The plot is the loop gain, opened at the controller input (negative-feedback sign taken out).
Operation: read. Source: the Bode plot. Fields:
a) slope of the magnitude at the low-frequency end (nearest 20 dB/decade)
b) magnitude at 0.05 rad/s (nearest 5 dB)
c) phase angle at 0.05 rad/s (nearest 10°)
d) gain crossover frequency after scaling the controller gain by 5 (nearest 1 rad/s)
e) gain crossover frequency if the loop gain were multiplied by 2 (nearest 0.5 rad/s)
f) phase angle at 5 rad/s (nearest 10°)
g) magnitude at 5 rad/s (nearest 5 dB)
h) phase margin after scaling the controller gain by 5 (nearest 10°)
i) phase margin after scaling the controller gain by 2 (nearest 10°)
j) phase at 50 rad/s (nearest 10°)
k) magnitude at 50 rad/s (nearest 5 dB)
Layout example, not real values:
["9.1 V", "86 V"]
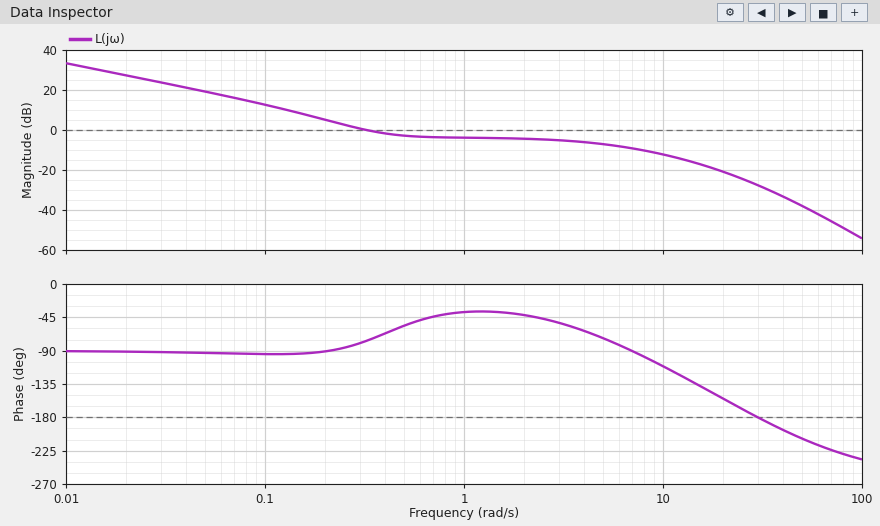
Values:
["-20 dB/decade", "20 dB", "-90°", "12 rad/s", "4.0 rad/s", "-70°", "-5 dB", "60°", "120°", "-210°", "-40 dB"]
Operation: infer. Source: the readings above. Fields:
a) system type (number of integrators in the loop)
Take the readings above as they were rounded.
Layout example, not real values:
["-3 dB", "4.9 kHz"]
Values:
["1"]
